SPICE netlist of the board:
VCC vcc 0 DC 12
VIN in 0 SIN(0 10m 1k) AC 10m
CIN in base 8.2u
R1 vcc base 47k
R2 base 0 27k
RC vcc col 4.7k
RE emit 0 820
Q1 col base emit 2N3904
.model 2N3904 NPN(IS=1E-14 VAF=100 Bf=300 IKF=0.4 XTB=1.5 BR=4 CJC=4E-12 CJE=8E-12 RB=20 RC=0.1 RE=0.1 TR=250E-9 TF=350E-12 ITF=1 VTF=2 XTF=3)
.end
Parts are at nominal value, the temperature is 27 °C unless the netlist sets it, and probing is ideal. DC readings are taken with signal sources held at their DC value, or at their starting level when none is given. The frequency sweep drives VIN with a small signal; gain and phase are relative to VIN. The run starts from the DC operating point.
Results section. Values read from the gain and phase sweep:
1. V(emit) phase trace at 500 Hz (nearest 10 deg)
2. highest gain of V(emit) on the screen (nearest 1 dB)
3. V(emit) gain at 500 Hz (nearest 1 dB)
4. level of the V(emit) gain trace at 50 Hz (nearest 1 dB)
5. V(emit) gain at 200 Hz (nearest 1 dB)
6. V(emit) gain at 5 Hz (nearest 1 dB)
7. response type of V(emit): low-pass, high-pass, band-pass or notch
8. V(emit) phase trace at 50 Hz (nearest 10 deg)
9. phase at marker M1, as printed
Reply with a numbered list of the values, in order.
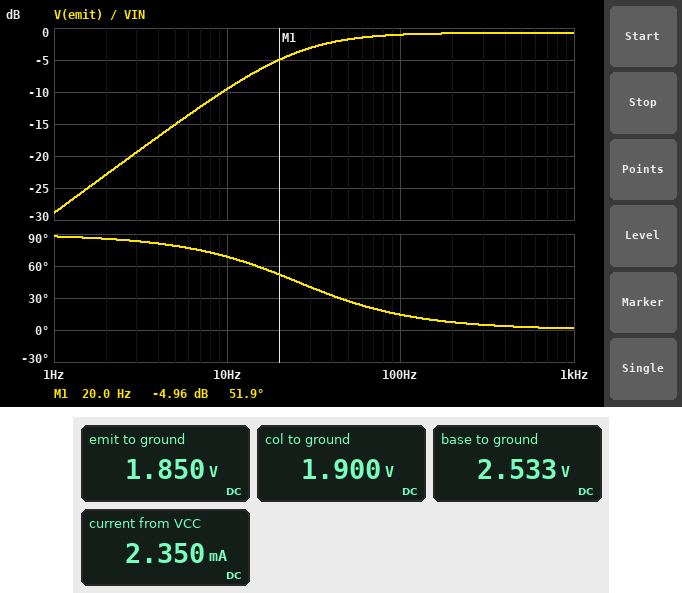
1. 0 deg
2. -1 dB
3. -1 dB
4. -2 dB
5. -1 dB
6. -15 dB
7. high-pass
8. 30 deg
9. 51.9 deg
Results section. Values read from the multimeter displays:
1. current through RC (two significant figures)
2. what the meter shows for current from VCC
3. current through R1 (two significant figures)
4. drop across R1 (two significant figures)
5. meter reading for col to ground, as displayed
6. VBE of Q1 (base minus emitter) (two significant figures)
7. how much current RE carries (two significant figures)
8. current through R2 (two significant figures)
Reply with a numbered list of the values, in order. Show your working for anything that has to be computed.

1. (12 V - 1.9 V) / 4.7 kΩ = 2.1 mA
2. 2.350 mA
3. (12 V - 2.533 V) / 47 kΩ = 200 µA
4. 12 V - 2.533 V = 9.5 V
5. 1.900 V
6. 2.533 V - 1.85 V = 680 mV
7. (1.85 V) / 820 Ω = 2.3 mA
8. (2.533 V) / 27 kΩ = 94 µA
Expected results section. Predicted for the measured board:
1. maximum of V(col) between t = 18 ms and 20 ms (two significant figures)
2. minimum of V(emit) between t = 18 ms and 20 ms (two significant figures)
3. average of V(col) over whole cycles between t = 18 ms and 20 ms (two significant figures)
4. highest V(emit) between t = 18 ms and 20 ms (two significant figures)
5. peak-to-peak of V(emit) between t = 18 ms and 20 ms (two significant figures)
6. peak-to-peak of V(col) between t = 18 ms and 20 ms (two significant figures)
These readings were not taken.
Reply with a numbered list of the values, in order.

1. 1.9 V
2. 1.8 V
3. 1.9 V
4. 1.9 V
5. 18 mV
6. 13 mV
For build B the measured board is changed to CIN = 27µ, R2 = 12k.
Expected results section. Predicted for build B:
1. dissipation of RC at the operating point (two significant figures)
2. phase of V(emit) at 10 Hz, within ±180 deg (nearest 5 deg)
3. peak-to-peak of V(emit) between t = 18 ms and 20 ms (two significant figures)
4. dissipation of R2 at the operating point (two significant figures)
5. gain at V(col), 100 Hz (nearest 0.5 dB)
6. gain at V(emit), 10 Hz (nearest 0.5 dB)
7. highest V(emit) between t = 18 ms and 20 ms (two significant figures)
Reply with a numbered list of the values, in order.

1. 20 mW
2. 5 deg
3. 20 mV
4. 470 µW
5. 15.0 dB
6. 0 dB
7. 1.7 V
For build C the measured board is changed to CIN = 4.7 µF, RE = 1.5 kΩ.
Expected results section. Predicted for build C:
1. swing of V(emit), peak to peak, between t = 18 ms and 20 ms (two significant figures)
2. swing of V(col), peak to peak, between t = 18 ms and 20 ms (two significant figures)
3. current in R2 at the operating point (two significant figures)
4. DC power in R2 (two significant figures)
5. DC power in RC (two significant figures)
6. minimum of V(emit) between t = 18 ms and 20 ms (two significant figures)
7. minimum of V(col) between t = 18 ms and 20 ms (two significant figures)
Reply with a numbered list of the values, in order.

1. 19 mV
2. 9.7 mV
3. 130 µA
4. 480 µW
5. 17 mW
6. 2.9 V
7. 3.0 V
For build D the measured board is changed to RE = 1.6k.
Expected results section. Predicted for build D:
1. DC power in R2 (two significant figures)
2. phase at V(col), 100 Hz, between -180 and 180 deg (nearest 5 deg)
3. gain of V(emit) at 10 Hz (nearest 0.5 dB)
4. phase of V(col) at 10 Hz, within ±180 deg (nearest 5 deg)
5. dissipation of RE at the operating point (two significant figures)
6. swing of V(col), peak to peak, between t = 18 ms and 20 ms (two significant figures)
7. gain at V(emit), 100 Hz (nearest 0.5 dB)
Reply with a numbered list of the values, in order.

1. 520 µW
2. 10 deg
3. -5.5 dB
4. 55 deg
5. 5.9 mW
6. 8.1 mV
7. -0.5 dB
